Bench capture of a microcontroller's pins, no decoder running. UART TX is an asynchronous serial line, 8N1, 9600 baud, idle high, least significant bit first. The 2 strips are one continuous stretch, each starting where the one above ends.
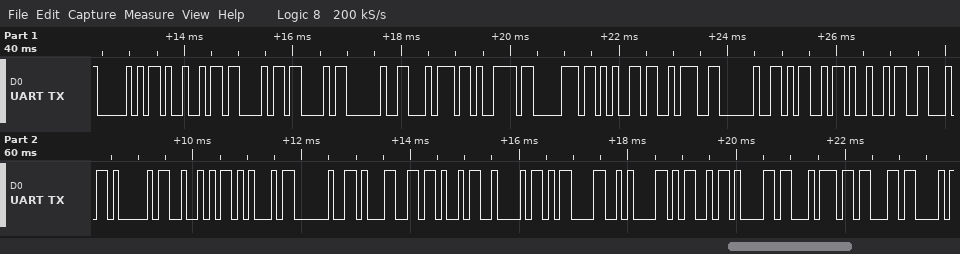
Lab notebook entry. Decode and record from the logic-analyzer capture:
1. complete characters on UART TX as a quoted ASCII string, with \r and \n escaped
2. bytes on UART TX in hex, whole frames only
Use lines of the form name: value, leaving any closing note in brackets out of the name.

complete characters on UART TX as a quoted ASCII string, with \r and \n escaped: "PICC type: MIFARE 1KB\r\nMatc"
bytes on UART TX in hex, whole frames only: 0x50 0x49 0x43 0x43 0x20 0x74 0x79 0x70 0x65 0x3A 0x20 0x4D 0x49 0x46 0x41 0x52 0x45 0x20 0x31 0x4B 0x42 0x0D 0x0A 0x4D 0x61 0x74 0x63
